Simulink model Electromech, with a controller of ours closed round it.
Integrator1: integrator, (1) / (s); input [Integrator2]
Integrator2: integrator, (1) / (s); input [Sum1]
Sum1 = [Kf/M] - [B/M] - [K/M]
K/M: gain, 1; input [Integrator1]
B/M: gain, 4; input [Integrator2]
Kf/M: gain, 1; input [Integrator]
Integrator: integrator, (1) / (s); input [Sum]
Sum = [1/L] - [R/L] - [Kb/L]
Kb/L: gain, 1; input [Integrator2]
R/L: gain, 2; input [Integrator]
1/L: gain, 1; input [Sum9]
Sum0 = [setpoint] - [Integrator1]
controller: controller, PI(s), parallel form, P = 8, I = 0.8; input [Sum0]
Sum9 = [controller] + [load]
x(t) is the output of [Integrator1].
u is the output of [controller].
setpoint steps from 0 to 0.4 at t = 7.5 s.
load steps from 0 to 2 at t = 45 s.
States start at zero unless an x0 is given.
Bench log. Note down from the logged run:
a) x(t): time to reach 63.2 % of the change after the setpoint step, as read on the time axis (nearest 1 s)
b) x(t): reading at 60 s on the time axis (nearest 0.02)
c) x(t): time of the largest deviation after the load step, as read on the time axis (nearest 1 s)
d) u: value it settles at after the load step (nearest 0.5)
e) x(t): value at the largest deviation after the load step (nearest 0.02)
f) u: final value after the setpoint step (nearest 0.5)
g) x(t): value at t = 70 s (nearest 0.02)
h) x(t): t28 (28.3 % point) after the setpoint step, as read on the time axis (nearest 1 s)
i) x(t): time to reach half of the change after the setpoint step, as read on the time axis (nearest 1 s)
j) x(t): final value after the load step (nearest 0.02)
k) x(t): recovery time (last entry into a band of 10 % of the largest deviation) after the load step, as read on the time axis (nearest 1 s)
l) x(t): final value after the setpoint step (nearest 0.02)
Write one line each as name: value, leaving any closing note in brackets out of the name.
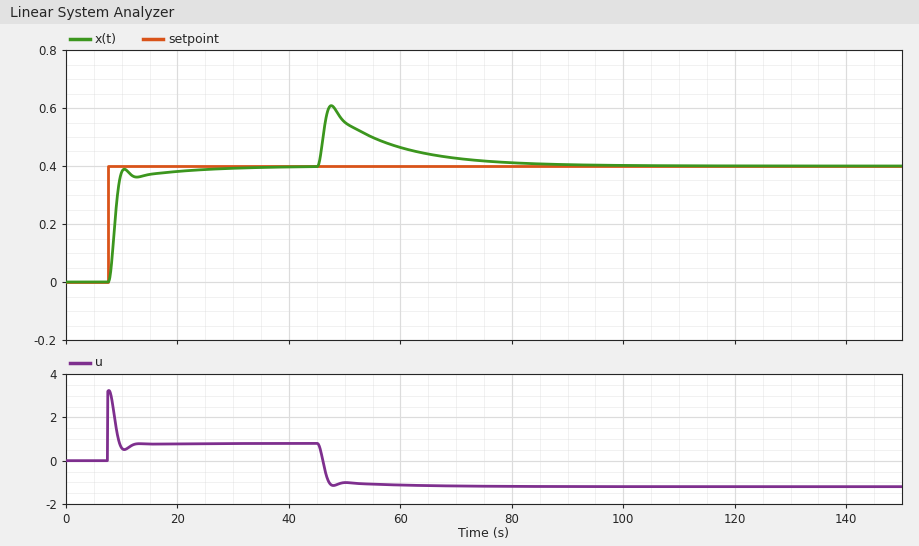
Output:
x(t): time to reach 63.2 % of the change after the setpoint step, as read on the time axis: 9 s
x(t): reading at 60 s on the time axis: 0.46
x(t): time of the largest deviation after the load step, as read on the time axis: 48 s
u: value it settles at after the load step: -1.0
x(t): value at the largest deviation after the load step: 0.60
u: final value after the setpoint step: 1.0
x(t): value at t = 70 s: 0.42
x(t): t28 (28.3 % point) after the setpoint step, as read on the time axis: 8 s
x(t): time to reach half of the change after the setpoint step, as read on the time axis: 9 s
x(t): final value after the load step: 0.40
x(t): recovery time (last entry into a band of 10 % of the largest deviation) after the load step, as read on the time axis: 73 s
x(t): final value after the setpoint step: 0.40
